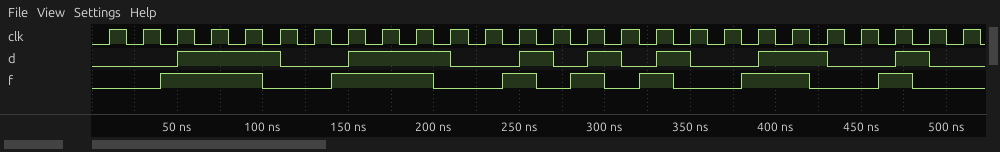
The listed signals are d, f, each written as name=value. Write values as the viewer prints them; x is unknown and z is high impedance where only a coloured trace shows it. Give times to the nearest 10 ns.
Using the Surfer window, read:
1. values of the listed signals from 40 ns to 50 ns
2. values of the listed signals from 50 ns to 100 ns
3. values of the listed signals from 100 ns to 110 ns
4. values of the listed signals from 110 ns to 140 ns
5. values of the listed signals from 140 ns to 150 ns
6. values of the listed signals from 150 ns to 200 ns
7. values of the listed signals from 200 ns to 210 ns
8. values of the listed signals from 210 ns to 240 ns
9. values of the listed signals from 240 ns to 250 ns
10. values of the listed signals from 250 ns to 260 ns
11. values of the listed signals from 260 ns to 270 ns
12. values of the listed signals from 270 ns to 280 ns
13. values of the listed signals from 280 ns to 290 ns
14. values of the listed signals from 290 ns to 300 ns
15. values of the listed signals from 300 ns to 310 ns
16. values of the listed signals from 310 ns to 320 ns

d=0, f=1
d=1, f=1
d=1, f=0
d=0, f=0
d=0, f=1
d=1, f=1
d=1, f=0
d=0, f=0
d=0, f=1
d=1, f=1
d=1, f=0
d=0, f=0
d=0, f=1
d=1, f=1
d=1, f=0
d=0, f=0
